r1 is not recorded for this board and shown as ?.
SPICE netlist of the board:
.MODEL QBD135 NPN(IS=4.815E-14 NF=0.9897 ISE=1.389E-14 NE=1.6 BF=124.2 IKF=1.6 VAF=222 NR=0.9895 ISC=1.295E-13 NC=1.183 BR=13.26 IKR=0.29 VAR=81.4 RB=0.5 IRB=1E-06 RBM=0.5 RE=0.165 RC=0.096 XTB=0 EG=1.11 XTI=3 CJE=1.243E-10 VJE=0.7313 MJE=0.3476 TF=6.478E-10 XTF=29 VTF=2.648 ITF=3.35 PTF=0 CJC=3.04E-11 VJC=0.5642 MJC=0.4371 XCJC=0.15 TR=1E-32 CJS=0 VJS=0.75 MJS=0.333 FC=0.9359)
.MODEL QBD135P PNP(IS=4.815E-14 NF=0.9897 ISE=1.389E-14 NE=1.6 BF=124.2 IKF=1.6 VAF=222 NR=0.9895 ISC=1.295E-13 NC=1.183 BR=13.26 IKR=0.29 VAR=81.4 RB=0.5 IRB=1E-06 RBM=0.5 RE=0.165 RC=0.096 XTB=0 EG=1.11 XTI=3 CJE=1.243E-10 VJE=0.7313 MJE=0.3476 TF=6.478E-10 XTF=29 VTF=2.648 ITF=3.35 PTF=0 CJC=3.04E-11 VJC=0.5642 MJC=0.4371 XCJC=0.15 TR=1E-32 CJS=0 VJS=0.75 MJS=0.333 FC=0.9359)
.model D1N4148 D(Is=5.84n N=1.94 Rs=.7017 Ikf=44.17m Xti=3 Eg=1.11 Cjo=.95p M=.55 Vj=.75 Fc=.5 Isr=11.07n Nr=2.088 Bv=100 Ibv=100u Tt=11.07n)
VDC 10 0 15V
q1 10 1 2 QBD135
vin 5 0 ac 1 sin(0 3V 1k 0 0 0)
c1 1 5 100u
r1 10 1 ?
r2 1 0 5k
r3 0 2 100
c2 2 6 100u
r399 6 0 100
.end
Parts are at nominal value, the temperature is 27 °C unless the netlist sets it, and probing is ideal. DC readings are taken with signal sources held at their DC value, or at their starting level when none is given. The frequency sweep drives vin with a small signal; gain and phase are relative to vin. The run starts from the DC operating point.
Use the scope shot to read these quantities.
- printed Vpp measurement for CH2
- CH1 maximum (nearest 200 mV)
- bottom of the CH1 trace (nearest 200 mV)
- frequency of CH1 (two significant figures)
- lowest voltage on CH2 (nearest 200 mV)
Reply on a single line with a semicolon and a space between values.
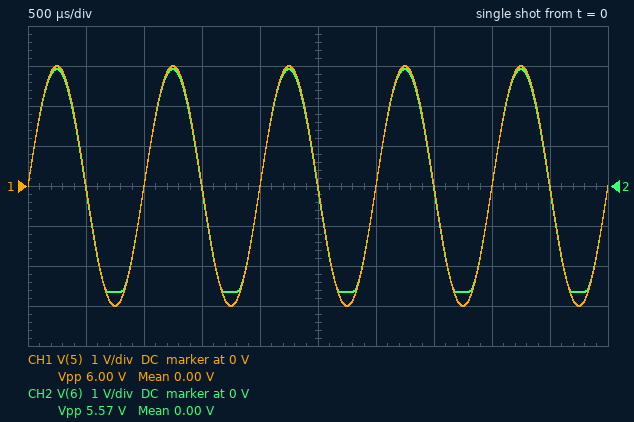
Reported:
5.57 V; 3.0 V; -3.0 V; 1.0 kHz; -2.6 V
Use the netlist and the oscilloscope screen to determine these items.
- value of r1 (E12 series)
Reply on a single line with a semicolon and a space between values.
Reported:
5.6 kΩ
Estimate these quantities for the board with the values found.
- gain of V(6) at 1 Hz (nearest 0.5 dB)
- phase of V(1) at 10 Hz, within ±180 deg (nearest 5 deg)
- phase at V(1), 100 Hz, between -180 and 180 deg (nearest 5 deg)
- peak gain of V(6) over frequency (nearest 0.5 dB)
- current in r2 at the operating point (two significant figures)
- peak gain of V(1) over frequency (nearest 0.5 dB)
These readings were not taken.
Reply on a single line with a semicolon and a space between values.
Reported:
-26.0 dB; 5 deg; 0 deg; 0 dB; 1.2 mA; 0 dB
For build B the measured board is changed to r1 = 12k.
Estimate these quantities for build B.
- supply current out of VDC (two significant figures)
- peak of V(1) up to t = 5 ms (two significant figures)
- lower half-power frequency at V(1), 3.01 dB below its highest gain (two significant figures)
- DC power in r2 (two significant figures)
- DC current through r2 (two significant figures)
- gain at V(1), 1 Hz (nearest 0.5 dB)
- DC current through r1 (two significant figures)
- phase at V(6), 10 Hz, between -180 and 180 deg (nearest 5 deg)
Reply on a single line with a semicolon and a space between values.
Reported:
30 mA; 6.6 V; 580 mHz; 2.6 mW; 720 µA; -1.5 dB; 950 µA; 60 deg
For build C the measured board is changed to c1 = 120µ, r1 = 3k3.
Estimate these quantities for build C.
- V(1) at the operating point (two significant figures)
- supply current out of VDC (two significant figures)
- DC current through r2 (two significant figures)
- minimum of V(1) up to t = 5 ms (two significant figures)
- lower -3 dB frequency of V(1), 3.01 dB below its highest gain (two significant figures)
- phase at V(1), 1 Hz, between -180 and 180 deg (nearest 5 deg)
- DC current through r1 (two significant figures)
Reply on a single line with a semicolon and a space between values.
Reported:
7.9 V; 73 mA; 1.6 mA; 4.9 V; 790 mHz; 40 deg; 2.2 mA
